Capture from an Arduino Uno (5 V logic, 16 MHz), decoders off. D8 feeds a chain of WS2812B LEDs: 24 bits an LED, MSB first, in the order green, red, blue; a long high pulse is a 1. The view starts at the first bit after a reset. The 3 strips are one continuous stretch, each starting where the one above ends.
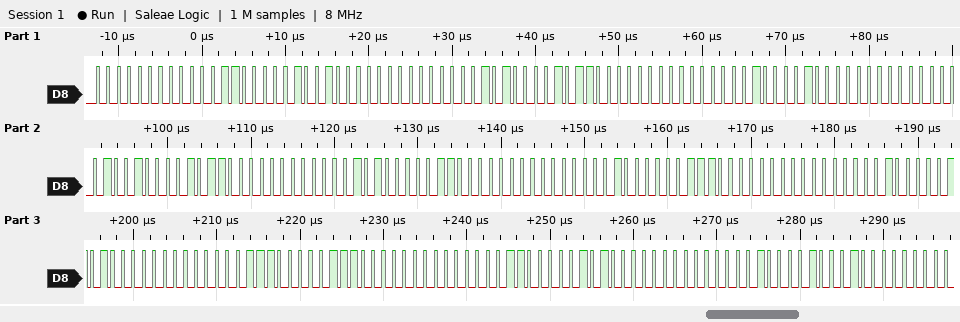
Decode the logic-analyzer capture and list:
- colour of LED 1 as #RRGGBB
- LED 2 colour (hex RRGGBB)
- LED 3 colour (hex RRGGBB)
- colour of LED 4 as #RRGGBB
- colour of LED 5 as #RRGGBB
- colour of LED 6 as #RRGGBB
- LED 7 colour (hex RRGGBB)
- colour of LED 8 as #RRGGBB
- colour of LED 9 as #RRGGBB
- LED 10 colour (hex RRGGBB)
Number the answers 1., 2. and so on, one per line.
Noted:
1. #0C0012
2. #05000B
3. #010008
4. #09000B
5. #0A000C
6. #04000E
7. #010005
8. #070007
9. #030005
10. #020011
